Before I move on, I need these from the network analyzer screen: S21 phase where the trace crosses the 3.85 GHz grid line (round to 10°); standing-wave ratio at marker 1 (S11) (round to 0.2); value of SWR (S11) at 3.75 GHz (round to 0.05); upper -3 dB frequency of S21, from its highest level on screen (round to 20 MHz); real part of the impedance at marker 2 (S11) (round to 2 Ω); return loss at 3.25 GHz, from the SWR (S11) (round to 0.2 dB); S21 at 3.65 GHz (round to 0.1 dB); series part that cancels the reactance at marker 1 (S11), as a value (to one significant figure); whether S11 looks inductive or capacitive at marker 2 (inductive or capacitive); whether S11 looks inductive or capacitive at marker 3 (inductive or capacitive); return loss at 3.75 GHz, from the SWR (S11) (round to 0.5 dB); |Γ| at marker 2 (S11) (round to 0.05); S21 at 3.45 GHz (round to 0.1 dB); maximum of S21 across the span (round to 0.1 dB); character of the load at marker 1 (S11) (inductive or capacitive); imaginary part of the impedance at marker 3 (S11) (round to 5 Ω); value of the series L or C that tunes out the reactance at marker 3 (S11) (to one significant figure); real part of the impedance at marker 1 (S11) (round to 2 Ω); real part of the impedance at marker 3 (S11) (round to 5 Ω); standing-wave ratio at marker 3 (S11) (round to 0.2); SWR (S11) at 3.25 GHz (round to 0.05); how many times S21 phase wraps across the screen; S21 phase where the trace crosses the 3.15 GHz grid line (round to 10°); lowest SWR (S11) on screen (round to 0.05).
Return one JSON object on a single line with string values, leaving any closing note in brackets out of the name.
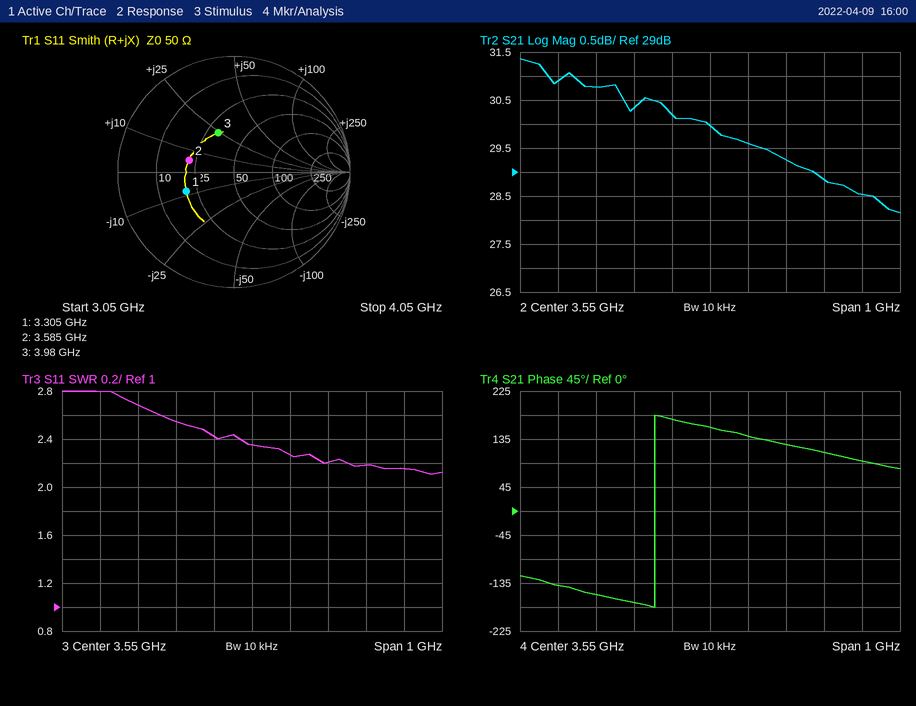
{"S21 phase where the trace crosses the 3.85 GHz grid line": "110°", "standing-wave ratio at marker 1 (S11)": "2.6", "value of SWR (S11) at 3.75 GHz": "2.20", "upper -3 dB frequency of S21, from its highest level on screen": "4.00 GHz", "real part of the impedance at marker 2 (S11)": "22 Ω", "return loss at 3.25 GHz, from the SWR (S11)": "6.8 dB", "S21 at 3.65 GHz": "29.6 dB", "series part that cancels the reactance at marker 1 (S11), as a value": "400 pH", "whether S11 looks inductive or capacitive at marker 2": "inductive", "whether S11 looks inductive or capacitive at marker 3": "inductive", "return loss at 3.75 GHz, from the SWR (S11)": "8.5 dB", "|Γ| at marker 2 (S11)": "0.40", "S21 at 3.45 GHz": "30.2 dB", "maximum of S21 across the span": "31.4 dB", "character of the load at marker 1 (S11)": "capacitive", "imaginary part of the impedance at marker 3 (S11)": "+25 Ω", "value of the series L or C that tunes out the reactance at marker 3 (S11)": "2 pF", "real part of the impedance at marker 1 (S11)": "20 Ω", "real part of the impedance at marker 3 (S11)": "30 Ω", "standing-wave ratio at marker 3 (S11)": "2.2", "SWR (S11) at 3.25 GHz": "2.70", "how many times S21 phase wraps across the screen": "1", "S21 phase where the trace crosses the 3.15 GHz grid line": "-140°", "lowest SWR (S11) on screen": "2.10"}
